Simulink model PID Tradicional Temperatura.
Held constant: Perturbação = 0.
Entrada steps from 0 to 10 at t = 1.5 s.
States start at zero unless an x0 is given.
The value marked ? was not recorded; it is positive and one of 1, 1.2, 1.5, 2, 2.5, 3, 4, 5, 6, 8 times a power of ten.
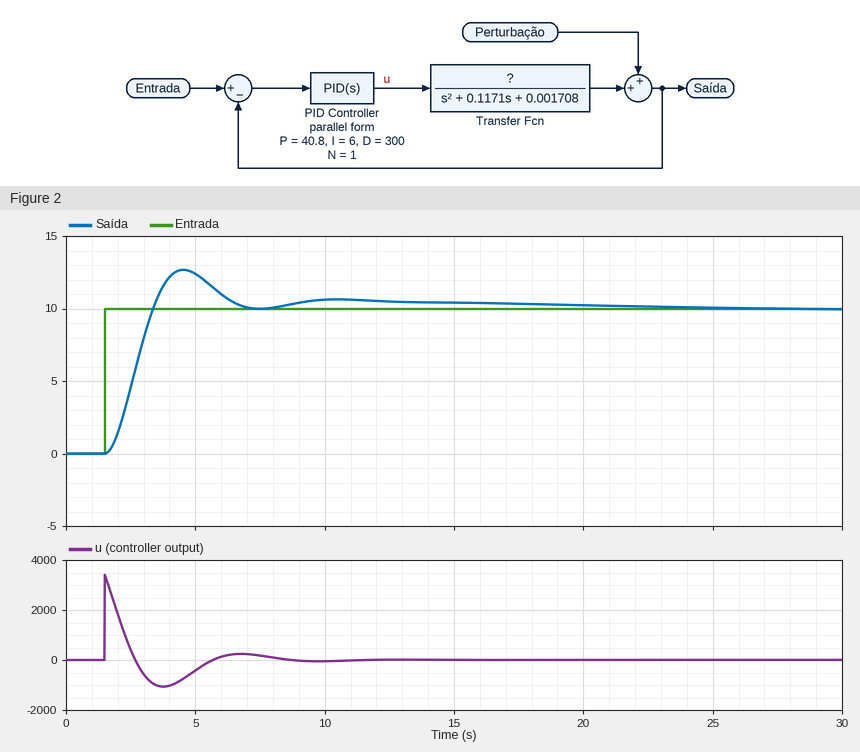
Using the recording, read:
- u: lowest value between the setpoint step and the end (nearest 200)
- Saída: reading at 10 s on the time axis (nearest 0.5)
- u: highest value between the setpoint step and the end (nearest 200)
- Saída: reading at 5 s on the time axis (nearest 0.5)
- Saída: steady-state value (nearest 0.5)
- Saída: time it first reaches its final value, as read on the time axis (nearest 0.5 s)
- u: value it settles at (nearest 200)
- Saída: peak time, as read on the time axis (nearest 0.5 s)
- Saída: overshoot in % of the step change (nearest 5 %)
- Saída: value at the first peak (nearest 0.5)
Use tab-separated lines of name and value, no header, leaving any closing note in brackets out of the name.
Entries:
u: lowest value between the setpoint step and the end	-1000
Saída: reading at 10 s on the time axis	10.5
u: highest value between the setpoint step and the end	3400
Saída: reading at 5 s on the time axis	12.5
Saída: steady-state value	10.0
Saída: time it first reaches its final value, as read on the time axis	3.5 s
u: value it settles at	0
Saída: peak time, as read on the time axis	4.5 s
Saída: overshoot in % of the step change	25 %
Saída: value at the first peak	12.5
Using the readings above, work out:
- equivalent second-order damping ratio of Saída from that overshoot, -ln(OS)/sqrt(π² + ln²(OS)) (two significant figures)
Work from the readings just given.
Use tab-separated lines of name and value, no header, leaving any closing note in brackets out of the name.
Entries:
equivalent second-order damping ratio of Saída from that overshoot, -ln(OS)/sqrt(π² + ln²(OS))	0.40
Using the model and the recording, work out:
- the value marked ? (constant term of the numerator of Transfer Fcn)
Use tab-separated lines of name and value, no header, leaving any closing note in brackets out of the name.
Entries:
the value marked ?	0.004
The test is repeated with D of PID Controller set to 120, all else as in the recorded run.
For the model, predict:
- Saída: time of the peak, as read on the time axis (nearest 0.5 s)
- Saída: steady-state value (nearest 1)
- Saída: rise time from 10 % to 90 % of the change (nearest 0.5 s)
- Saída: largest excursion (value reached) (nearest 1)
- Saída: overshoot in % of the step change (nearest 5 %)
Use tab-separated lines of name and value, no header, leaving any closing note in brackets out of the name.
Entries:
Saída: time of the peak, as read on the time axis	6.5 s
Saída: steady-state value	10
Saída: rise time from 10 % to 90 % of the change	2.0 s
Saída: largest excursion (value reached)	14
Saída: overshoot in % of the step change	40 %
